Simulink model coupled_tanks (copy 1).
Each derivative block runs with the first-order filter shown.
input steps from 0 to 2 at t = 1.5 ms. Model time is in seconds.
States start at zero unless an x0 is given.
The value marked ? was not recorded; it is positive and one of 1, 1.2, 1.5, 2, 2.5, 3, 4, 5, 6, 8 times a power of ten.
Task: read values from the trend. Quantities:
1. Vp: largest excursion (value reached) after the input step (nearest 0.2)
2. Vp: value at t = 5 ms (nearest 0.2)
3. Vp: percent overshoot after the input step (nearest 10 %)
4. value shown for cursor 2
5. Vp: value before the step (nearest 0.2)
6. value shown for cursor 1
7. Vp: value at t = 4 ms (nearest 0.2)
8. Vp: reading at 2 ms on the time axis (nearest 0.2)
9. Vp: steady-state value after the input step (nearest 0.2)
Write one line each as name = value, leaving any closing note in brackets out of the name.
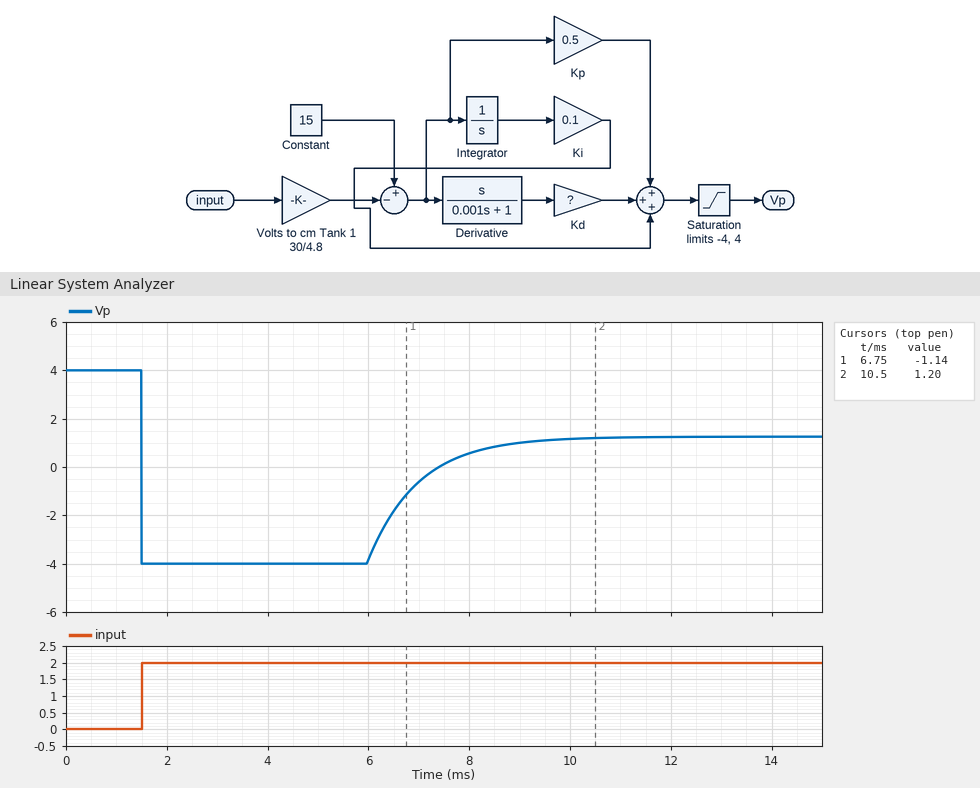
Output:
Vp: largest excursion (value reached) after the input step = -4.0
Vp: value at t = 5 ms = -4.0
Vp: percent overshoot after the input step = 190 %
value shown for cursor 2 = 1.20
Vp: value before the step = 4.0
value shown for cursor 1 = -1.14
Vp: value at t = 4 ms = -4.0
Vp: reading at 2 ms on the time axis = -4.0
Vp: steady-state value after the input step = 1.2
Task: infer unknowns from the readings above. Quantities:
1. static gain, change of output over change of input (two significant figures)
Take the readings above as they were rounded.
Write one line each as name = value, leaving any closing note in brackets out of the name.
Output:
static gain, change of output over change of input = -1.4
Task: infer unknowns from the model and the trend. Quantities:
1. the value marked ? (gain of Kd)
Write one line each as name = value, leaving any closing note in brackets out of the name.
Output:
the value marked ? = 0.05
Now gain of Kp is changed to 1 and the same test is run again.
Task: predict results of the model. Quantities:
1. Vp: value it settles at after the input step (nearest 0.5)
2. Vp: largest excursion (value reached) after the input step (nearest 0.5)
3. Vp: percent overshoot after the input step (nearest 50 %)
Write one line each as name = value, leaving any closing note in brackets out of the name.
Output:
Vp: value it settles at after the input step = 2.5
Vp: largest excursion (value reached) after the input step = -4.0
Vp: percent overshoot after the input step = 450 %
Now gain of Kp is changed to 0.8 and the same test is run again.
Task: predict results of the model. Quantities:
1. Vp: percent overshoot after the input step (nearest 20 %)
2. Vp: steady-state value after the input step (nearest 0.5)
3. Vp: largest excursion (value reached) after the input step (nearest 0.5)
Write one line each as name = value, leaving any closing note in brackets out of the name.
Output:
Vp: percent overshoot after the input step = 300 %
Vp: steady-state value after the input step = 2.0
Vp: largest excursion (value reached) after the input step = -4.0
